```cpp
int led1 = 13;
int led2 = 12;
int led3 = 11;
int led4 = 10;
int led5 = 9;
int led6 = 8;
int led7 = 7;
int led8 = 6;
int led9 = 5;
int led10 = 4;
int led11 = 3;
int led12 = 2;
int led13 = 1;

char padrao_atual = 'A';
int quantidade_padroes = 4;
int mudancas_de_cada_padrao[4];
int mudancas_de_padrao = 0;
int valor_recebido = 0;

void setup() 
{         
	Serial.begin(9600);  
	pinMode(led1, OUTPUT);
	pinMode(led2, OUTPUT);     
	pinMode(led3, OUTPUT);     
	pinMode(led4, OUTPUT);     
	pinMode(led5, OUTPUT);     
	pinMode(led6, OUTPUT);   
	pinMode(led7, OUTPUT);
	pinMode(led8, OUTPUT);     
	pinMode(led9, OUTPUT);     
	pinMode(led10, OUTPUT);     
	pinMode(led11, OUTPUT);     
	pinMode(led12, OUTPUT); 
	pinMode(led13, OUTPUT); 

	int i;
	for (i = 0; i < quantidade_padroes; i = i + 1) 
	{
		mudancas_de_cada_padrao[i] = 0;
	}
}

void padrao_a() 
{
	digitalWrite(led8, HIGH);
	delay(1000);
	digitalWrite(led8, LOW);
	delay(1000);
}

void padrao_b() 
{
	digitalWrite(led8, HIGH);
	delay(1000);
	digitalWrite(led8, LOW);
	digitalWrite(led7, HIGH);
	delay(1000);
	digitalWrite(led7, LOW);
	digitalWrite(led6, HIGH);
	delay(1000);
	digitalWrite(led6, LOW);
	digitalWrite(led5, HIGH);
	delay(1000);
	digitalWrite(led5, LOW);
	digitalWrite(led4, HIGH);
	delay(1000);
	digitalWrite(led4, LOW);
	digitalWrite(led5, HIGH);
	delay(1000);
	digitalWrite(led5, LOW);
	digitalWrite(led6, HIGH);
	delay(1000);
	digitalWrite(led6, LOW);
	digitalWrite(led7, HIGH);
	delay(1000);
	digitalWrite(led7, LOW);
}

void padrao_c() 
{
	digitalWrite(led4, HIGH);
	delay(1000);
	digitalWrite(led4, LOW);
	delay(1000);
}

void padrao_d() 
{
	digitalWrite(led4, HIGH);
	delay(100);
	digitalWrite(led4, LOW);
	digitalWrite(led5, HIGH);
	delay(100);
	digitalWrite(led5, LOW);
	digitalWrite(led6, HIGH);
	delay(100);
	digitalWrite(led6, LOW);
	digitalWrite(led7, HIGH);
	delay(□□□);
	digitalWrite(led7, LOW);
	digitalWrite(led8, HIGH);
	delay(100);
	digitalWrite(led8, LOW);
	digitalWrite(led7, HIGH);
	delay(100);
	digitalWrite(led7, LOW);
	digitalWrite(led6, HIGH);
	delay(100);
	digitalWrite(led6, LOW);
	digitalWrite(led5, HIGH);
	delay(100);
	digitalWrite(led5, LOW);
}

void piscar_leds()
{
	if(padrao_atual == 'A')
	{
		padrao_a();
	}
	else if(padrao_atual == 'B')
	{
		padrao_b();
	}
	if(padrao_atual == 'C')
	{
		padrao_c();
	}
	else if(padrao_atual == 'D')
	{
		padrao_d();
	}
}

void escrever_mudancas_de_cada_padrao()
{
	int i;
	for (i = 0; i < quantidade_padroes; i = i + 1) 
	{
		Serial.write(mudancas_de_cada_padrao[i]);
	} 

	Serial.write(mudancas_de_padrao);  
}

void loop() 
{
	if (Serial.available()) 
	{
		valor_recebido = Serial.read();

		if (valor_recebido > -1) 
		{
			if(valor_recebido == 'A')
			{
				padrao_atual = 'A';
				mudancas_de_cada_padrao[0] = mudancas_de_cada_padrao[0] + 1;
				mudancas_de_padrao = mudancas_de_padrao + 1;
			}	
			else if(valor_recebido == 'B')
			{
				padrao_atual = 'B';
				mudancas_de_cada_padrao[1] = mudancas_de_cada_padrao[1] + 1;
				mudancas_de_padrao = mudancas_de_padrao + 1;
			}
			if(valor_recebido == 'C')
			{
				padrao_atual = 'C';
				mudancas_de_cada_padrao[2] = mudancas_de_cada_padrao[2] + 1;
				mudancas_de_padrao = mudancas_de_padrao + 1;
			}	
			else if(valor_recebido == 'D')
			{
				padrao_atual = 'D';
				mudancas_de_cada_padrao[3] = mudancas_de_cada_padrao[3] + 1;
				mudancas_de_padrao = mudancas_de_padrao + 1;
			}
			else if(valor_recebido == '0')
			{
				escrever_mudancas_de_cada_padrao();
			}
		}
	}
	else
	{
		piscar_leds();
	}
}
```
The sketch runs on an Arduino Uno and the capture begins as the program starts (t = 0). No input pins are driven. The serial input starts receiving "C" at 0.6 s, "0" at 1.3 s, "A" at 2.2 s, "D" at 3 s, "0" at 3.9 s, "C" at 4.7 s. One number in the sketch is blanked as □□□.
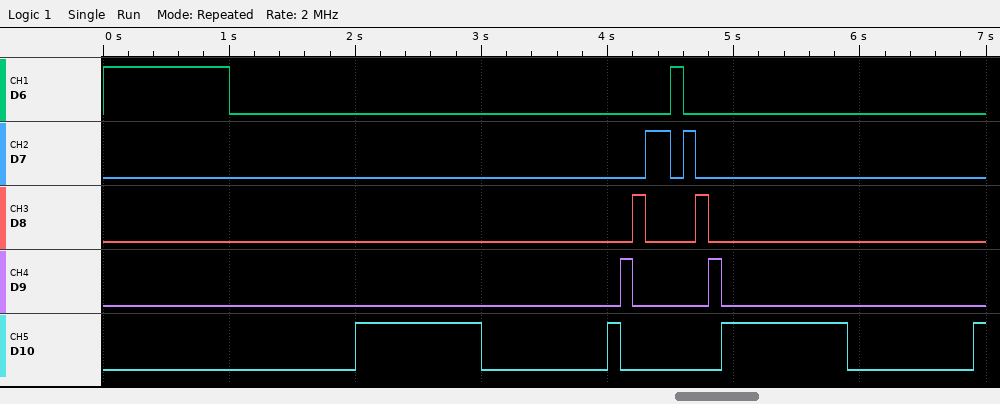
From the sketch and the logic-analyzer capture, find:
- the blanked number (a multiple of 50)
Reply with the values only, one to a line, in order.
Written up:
200
